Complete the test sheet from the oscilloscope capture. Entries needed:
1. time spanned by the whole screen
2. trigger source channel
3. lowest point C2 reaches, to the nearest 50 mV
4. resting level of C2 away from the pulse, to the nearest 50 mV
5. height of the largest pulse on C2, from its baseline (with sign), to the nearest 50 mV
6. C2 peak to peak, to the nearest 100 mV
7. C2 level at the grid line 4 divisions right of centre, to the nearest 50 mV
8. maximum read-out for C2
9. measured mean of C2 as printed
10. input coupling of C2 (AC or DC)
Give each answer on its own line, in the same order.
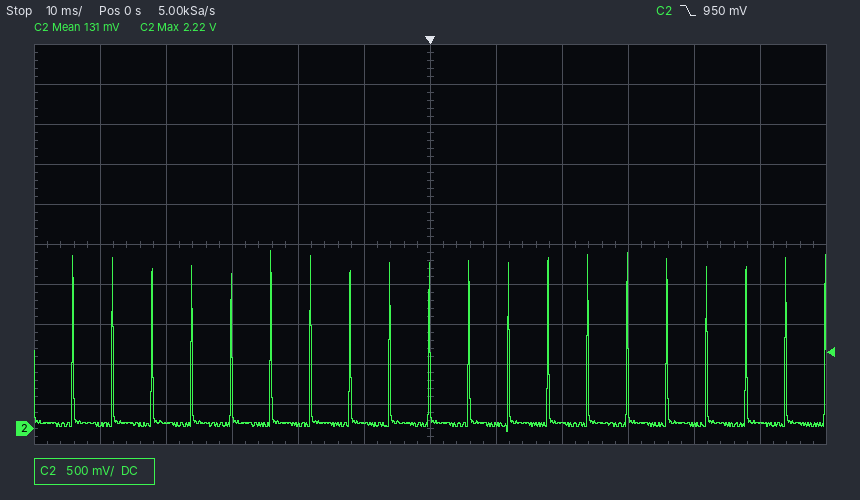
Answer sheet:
120 ms
C2
-50 mV
50 mV
+2.15 V
2.30 V
50 mV
2.22 V
131 mV
DC
